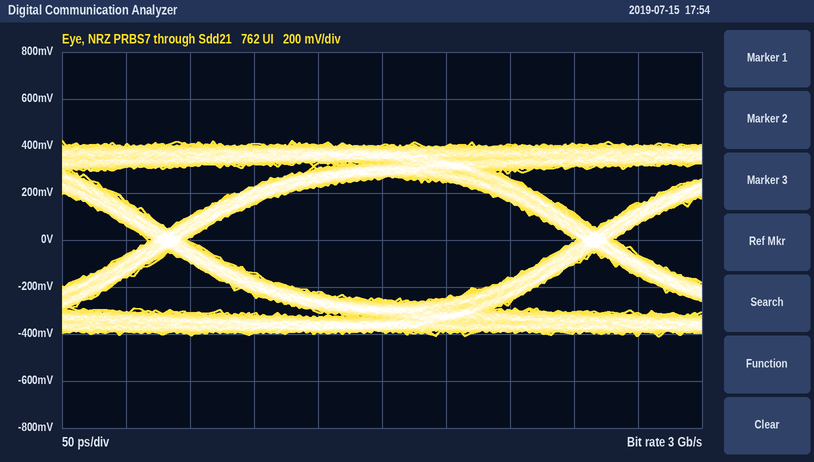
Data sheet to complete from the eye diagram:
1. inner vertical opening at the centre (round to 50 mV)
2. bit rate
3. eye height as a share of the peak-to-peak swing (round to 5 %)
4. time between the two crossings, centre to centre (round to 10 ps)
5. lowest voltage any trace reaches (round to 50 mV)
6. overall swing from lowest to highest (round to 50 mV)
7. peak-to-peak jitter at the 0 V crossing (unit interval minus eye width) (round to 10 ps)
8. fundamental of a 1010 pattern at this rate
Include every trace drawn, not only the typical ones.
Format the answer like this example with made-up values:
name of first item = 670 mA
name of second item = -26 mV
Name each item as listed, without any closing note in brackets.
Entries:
inner vertical opening at the centre = 500 mV
bit rate = 3 Gb/s
eye height as a share of the peak-to-peak swing = 60 %
time between the two crossings, centre to centre = 330 ps
lowest voltage any trace reaches = -400 mV
overall swing from lowest to highest = 850 mV
peak-to-peak jitter at the 0 V crossing (unit interval minus eye width) = 30 ps
fundamental of a 1010 pattern at this rate = 1.5 GHz
